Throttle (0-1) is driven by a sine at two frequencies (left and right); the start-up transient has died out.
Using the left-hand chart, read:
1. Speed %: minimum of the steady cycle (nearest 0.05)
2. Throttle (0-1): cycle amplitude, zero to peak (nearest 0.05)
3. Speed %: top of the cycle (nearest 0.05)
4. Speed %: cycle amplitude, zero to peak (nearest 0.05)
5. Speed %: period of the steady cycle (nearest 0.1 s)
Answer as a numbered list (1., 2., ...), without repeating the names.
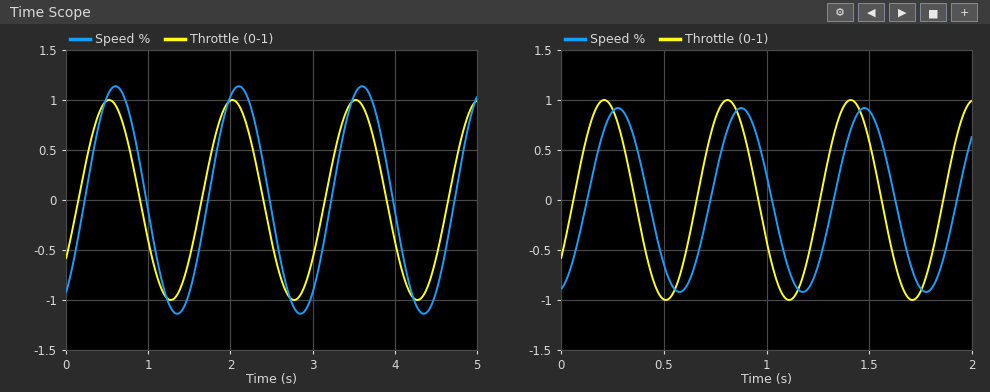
1. -1.15
2. 1.00
3. 1.15
4. 1.15
5. 1.5 s
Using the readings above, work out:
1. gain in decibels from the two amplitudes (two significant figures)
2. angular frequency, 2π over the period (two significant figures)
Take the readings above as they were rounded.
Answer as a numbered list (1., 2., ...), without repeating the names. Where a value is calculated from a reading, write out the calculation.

1. 20 log10(1.15 / 1) = 1.2 dB
2. 2π / 1.5 = 4.2 rad/s
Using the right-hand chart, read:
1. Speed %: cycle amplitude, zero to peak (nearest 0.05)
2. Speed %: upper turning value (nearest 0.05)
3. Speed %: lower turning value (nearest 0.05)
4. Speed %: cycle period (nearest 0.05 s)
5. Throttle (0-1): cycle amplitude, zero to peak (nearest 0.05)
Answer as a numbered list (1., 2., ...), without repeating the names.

1. 0.90
2. 0.90
3. -0.90
4. 0.60 s
5. 1.00
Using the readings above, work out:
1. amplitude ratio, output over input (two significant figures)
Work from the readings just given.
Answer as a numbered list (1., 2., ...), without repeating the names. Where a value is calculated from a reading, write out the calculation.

1. 0.9 / 1 = 0.90
